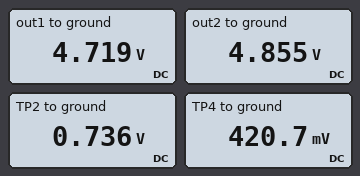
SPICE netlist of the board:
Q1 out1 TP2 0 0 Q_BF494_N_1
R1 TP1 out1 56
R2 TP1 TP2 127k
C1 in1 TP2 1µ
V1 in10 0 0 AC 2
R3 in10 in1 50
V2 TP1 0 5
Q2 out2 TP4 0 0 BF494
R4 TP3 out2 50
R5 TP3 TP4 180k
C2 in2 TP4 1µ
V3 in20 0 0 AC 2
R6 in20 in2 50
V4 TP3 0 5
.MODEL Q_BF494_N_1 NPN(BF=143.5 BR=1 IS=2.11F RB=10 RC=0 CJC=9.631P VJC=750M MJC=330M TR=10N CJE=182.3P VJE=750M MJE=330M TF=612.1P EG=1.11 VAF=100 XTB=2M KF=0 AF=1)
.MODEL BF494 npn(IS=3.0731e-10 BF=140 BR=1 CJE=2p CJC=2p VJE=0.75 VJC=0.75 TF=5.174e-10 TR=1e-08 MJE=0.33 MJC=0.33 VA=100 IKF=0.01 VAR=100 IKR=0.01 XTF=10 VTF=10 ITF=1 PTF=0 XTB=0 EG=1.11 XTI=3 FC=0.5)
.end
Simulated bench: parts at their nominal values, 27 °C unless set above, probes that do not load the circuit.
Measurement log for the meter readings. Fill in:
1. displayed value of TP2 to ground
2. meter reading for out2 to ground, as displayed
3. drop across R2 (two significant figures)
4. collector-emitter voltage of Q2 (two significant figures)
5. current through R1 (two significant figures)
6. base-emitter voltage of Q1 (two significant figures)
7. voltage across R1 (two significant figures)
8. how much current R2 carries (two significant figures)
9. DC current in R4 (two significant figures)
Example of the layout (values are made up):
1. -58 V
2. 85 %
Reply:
1. 0.736 V
2. 4.855 V
3. 4.3 V
4. 4.9 V
5. 5.0 mA
6. 740 mV
7. 280 mV
8. 34 µA
9. 2.9 mA
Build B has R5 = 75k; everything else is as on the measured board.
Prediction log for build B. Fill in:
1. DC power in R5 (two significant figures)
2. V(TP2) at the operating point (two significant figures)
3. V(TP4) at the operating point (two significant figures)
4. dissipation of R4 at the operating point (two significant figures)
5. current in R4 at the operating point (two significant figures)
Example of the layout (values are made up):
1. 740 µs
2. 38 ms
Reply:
1. 280 µW
2. 740 mV
3. 440 mV
4. 1.6 mW
5. 5.7 mA
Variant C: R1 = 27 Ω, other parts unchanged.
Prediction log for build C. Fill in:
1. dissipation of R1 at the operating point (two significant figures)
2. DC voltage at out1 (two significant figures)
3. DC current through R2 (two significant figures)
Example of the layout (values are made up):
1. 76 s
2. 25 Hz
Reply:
1. 680 µW
2. 4.9 V
3. 34 µA
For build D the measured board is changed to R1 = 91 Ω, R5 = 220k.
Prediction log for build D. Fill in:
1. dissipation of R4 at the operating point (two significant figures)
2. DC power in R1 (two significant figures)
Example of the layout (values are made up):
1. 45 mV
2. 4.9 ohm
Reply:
1. 300 µW
2. 2.3 mW
